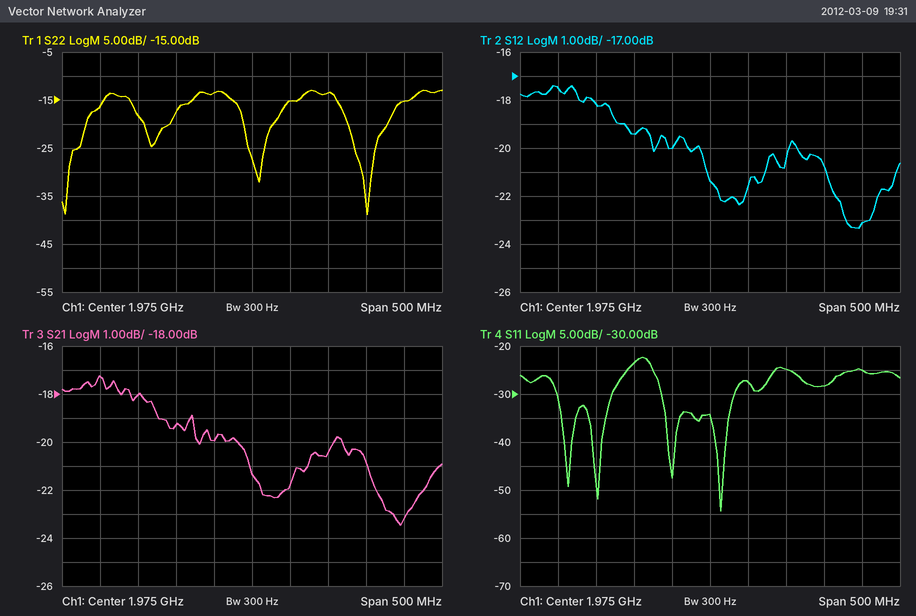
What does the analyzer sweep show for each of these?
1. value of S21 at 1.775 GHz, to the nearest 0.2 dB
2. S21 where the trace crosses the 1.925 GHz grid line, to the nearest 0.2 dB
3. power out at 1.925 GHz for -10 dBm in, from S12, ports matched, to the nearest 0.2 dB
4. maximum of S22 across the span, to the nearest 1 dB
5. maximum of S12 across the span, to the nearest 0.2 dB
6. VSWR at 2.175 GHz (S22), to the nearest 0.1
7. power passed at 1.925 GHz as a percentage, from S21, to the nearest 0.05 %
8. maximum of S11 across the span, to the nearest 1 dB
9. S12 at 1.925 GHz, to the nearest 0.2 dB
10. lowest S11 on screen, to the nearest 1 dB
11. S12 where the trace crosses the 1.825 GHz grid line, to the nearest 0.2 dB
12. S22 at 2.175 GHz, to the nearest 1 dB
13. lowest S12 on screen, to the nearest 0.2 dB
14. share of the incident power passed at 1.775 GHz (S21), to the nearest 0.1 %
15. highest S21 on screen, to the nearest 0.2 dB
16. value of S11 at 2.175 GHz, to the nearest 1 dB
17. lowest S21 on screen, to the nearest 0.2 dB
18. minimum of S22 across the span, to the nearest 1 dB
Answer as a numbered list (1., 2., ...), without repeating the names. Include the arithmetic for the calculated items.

1. -17.2 dB
2. -20.0 dB
3. -10 dBm + (-20.0 dB) = -30.0 dBm
4. -13 dB
5. -17.4 dB
6. |Γ| = 10^(-15/20) = 0.1778; VSWR = (1 + 0.1778)/(1 − 0.1778) ≈ 1.4
7. 10^(-20/10) ≈ 1.00 %
8. -22 dB
9. -20.0 dB
10. -54 dB
11. -18.2 dB
12. -15 dB
13. -23.4 dB
14. 10^(-17.2/10) ≈ 1.9 %
15. -17.2 dB
16. -25 dB
17. -23.4 dB
18. -39 dB
